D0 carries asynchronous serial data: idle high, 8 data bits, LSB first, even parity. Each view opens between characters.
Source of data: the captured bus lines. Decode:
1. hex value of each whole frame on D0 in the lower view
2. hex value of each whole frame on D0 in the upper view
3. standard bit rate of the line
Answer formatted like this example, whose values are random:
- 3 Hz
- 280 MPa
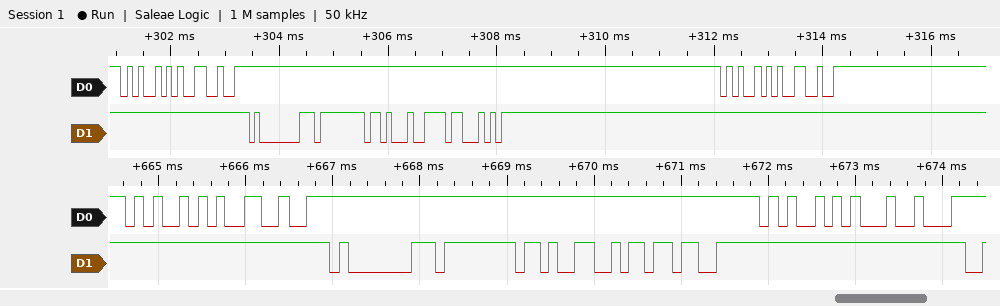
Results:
- A5, 26, A5, 24
- A5, 26, A5, 26
- 9600 baud
